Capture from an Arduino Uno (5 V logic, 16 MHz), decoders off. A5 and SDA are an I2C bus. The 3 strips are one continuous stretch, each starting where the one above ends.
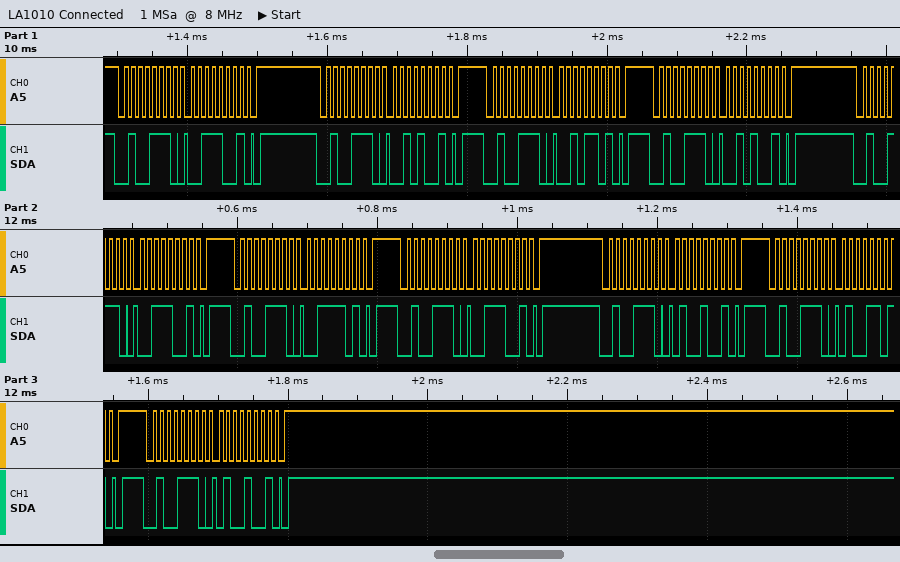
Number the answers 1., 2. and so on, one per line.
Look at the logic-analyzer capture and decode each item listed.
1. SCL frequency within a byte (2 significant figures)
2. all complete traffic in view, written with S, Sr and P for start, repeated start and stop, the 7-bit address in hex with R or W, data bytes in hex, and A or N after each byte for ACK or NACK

1. 100 kHz
2. S 27W A 39 A P S 27W A 29 A P S 27W A 2D A P S 27W A 29 A P S 27W A 39 A P S 27W A 3D A P S 27W A 39 A P S 27W A 49 A P S 27W A 4D A P S 27W A 49 A P
